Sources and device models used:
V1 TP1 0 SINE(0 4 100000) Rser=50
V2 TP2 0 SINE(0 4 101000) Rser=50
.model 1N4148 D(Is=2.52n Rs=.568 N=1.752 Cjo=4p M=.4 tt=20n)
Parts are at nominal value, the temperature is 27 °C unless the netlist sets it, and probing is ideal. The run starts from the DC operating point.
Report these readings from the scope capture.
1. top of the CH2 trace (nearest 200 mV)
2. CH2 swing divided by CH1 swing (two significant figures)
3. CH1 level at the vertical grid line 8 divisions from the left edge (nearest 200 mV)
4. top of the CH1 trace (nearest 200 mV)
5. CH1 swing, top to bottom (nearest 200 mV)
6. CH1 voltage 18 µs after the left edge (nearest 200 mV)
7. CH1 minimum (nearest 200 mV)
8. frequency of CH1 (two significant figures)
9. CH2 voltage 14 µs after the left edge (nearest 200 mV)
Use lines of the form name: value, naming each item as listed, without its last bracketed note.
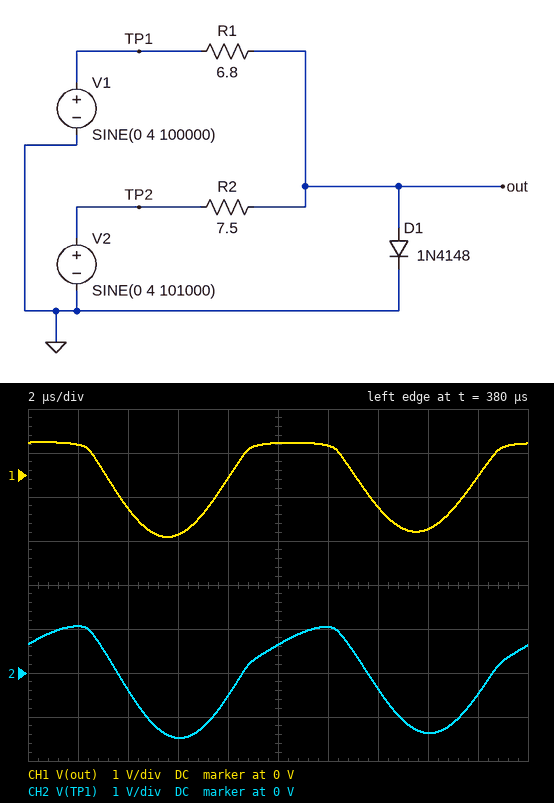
top of the CH2 trace: 1.0 V
CH2 swing divided by CH1 swing: 1.2
CH1 level at the vertical grid line 8 divisions from the left edge: -1.2 V
top of the CH1 trace: 800 mV
CH1 swing, top to bottom: 2.2 V
CH1 voltage 18 µs after the left edge: 0 V
CH1 minimum: -1.4 V
frequency of CH1: 100 kHz
CH2 voltage 14 µs after the left edge: -400 mV
